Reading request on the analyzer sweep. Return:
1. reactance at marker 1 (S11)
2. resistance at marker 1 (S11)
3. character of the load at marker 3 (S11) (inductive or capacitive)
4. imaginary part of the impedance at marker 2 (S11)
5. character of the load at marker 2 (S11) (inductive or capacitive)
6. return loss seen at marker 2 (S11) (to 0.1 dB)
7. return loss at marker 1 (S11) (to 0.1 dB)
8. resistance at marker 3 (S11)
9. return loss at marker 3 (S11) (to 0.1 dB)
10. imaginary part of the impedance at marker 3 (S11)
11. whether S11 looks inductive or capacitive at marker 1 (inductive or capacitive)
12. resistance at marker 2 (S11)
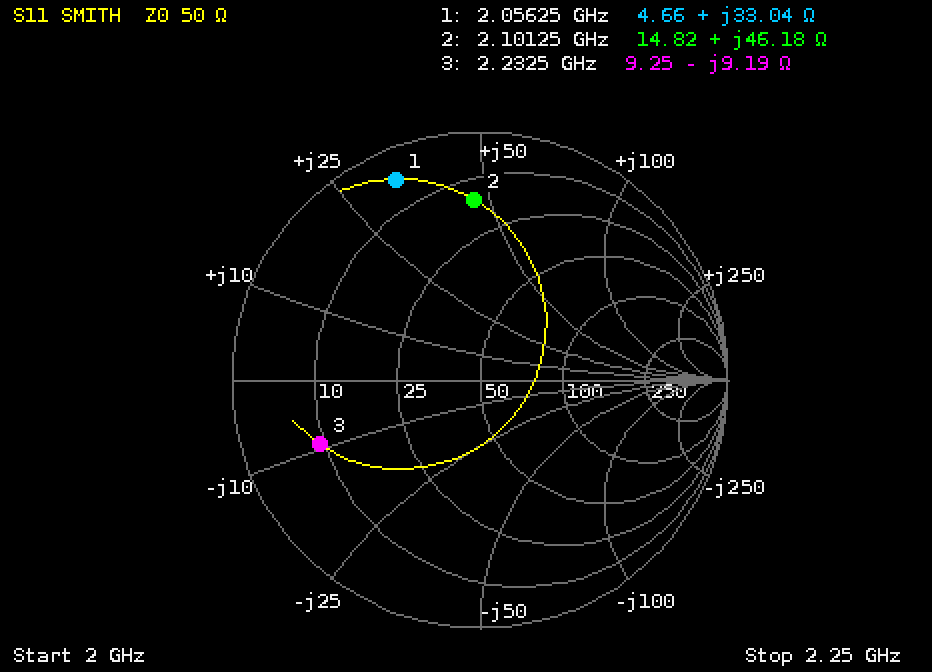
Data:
+33.04 Ω
4.66 Ω
capacitive
+46.18 Ω
inductive
2.7 dB
1.1 dB
9.25 Ω
3.1 dB
-9.19 Ω
inductive
14.82 Ω
